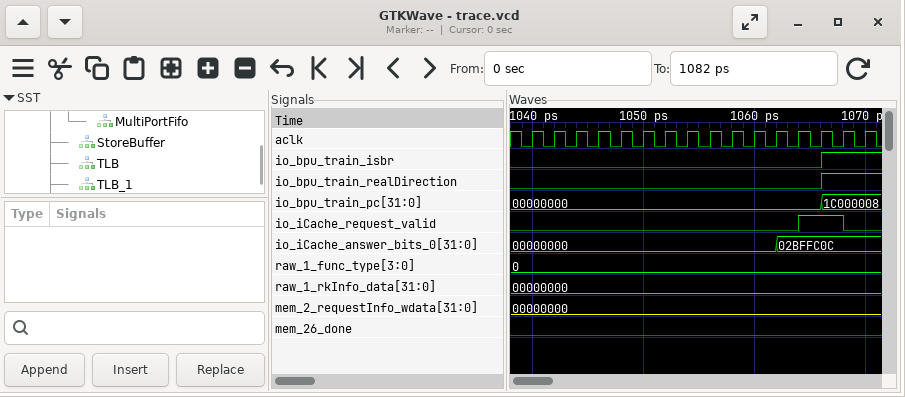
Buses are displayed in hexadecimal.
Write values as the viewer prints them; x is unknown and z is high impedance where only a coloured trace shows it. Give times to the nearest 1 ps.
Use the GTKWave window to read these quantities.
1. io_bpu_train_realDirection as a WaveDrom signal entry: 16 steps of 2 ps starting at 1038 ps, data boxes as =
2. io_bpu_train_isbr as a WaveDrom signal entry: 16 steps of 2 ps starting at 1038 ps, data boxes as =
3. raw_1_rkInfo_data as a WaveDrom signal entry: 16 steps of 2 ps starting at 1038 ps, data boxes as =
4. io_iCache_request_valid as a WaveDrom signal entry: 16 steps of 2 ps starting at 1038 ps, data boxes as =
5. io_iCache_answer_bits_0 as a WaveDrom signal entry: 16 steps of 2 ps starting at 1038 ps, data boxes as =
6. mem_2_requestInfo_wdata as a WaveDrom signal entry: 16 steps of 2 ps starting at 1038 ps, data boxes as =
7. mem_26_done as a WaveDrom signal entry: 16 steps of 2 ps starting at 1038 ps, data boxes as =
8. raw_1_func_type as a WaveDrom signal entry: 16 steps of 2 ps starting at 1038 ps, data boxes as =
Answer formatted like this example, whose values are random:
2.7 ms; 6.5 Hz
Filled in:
{name: 'io_bpu_train_realDirection', wave: '0.............1.'}; {name: 'io_bpu_train_isbr', wave: '0.............1.'}; {name: 'raw_1_rkInfo_data', wave: '=...............', data: '00000000'}; {name: 'io_iCache_request_valid', wave: '0............1.0'}; {name: 'io_iCache_answer_bits_0', wave: '=...........=...', data: '00000000 02BFFC0C'}; {name: 'mem_2_requestInfo_wdata', wave: '=...............', data: '00000000'}; {name: 'mem_26_done', wave: '0...............'}; {name: 'raw_1_func_type', wave: '=...............', data: '0'}
